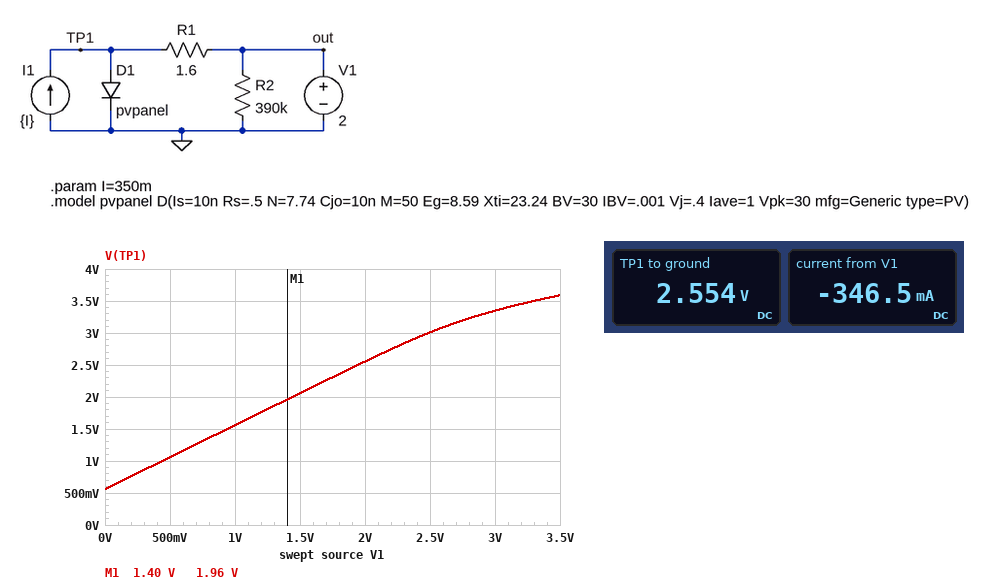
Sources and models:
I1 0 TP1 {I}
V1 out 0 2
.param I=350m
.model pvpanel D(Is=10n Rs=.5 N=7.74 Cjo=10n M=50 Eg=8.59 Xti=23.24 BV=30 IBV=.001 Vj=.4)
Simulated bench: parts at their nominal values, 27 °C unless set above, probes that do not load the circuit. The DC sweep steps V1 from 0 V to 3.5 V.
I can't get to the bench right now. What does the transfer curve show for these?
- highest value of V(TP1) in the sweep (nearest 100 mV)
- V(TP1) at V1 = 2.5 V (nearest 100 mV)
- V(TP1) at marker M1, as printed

3.6 V
3.0 V
1.96 V
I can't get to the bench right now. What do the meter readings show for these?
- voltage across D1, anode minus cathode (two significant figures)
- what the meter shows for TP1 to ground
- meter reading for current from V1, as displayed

2.6 V
2.554 V
-346.5 mA
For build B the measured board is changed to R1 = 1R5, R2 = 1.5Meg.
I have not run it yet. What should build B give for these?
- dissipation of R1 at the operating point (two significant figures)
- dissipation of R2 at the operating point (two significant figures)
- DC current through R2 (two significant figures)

180 mW
2.7 µW
1.3 µA
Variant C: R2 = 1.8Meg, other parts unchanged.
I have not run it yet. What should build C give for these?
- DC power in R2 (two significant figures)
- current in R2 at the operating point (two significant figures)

2.2 µW
1.1 µA
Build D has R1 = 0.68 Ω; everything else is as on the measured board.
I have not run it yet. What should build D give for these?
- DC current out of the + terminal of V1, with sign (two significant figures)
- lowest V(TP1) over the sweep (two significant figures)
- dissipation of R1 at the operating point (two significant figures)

-350 mA
240 mV
83 mW
